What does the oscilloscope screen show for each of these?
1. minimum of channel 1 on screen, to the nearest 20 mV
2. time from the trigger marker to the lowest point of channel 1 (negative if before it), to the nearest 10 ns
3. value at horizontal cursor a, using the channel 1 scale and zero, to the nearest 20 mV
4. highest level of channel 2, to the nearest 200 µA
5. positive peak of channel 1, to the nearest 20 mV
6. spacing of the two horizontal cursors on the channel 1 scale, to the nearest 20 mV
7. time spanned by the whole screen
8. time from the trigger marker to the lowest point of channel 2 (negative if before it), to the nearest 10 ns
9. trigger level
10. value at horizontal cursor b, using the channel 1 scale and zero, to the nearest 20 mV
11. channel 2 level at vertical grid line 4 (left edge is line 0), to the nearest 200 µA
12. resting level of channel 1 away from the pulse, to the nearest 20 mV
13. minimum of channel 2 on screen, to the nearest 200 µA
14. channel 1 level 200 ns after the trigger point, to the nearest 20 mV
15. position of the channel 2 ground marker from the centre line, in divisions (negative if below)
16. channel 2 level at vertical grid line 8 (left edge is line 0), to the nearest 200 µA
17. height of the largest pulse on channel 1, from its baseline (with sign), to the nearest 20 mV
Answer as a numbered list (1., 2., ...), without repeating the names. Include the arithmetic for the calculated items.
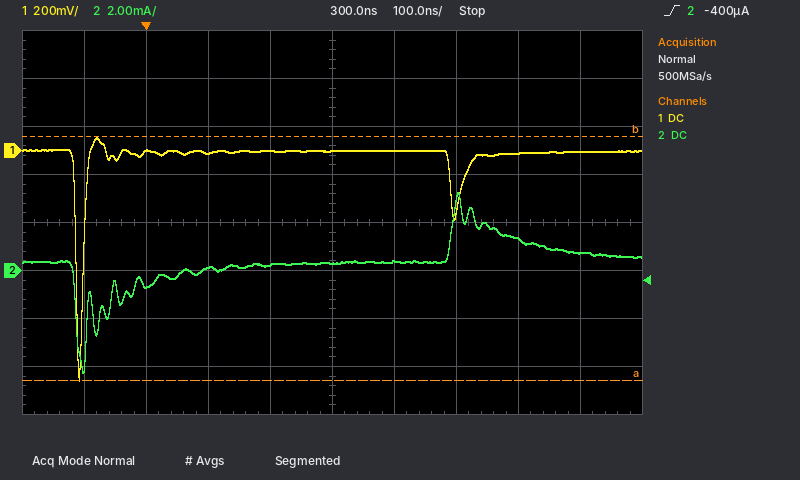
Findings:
1. -960 mV
2. -110 ns
3. -960 mV
4. 3.2 mA
5. 60 mV
6. 1.02 V
7. 1 µs
8. -100 ns
9. -400 µA
10. 60 mV
11. 200 µA
12. 0 mV
13. -4.2 mA
14. 0 mV
15. -1.0 div
16. 1.4 mA
17. -960 mV − (0 mV) = -960 mV
